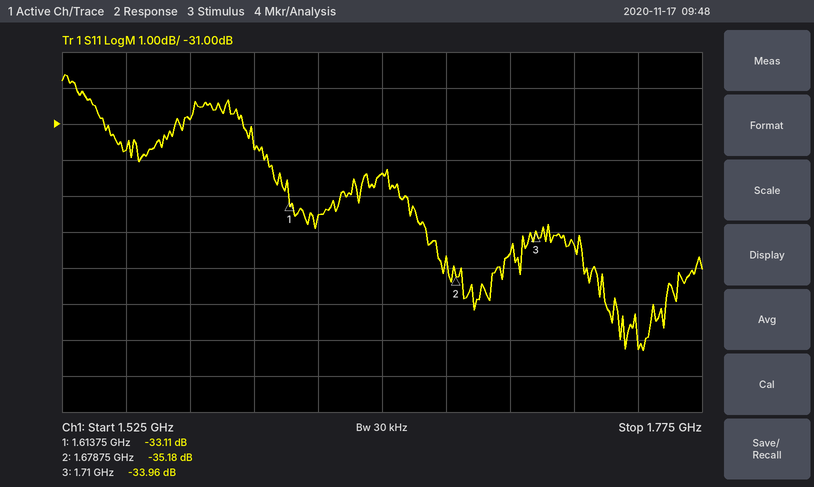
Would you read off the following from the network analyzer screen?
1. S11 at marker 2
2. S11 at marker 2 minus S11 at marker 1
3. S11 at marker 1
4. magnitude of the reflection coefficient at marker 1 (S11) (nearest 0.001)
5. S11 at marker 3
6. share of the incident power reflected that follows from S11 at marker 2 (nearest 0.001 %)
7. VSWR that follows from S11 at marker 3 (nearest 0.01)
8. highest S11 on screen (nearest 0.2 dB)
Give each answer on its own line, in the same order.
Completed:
-35.18 dB
-2.07 dB
-33.11 dB
0.022
-33.96 dB
0.030 %
1.04
-29.6 dB
